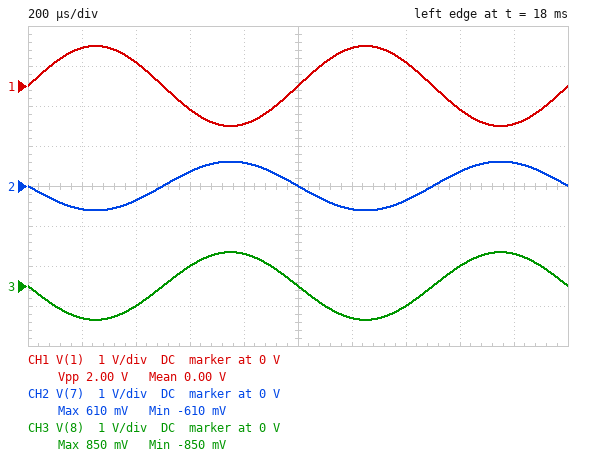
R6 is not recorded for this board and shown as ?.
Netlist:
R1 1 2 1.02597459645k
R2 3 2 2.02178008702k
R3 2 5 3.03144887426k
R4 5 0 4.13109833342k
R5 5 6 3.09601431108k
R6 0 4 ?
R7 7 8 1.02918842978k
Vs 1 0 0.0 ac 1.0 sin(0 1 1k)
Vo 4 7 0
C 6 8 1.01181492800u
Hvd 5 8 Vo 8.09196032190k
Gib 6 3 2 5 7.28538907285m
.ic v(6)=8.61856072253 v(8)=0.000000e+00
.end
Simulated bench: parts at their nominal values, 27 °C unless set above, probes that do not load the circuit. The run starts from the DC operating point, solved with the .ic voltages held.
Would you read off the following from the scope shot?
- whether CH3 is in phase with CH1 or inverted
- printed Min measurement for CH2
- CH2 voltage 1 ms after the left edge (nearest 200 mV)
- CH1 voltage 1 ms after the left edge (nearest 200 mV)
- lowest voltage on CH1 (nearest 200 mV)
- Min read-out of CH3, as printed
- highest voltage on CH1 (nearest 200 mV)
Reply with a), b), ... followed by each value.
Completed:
a) inverted
b) -610 mV
c) 0 V
d) 0 V
e) -1.0 V
f) -850 mV
g) 1.0 V
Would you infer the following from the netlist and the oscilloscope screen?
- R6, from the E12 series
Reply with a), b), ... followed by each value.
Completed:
a) 2.7 kΩ
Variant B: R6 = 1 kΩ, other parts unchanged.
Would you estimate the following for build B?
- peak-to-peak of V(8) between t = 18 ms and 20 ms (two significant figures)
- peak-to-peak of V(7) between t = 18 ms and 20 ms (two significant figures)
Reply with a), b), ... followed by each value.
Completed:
a) 630 mV
b) 310 mV
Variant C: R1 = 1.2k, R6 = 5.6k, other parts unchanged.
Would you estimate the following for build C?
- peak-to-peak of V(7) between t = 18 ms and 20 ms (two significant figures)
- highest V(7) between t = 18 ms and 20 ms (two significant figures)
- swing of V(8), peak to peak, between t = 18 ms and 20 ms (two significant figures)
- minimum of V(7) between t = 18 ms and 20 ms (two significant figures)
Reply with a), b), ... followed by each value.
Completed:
a) 14 V
b) 7.2 V
c) 17 V
d) -7.2 V
